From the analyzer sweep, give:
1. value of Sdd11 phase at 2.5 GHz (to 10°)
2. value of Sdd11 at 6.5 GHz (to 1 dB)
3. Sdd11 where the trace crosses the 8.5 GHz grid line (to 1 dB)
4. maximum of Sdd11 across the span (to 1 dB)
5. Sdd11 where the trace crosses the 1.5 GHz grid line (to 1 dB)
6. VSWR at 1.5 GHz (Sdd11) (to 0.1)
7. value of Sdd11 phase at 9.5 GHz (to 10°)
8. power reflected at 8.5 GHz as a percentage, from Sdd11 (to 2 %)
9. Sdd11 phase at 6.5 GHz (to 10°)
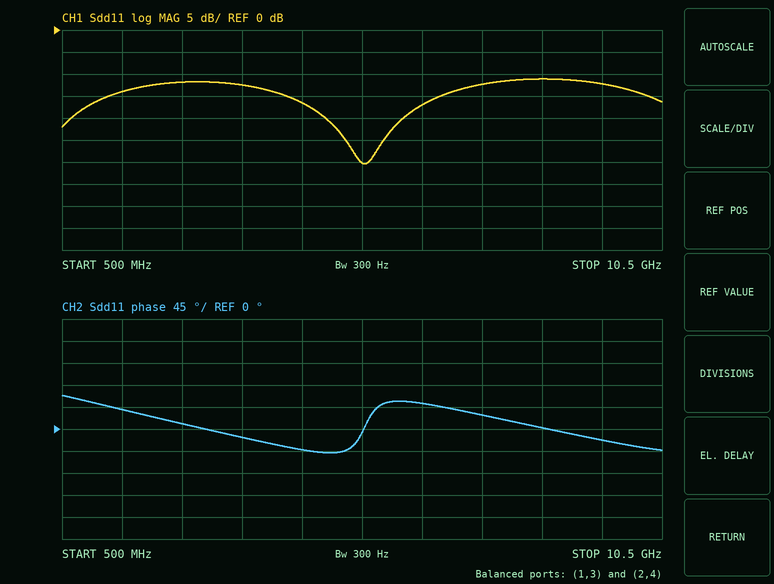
10°
-17 dB
-11 dB
-11 dB
-14 dB
1.5
-20°
8 %
50°
